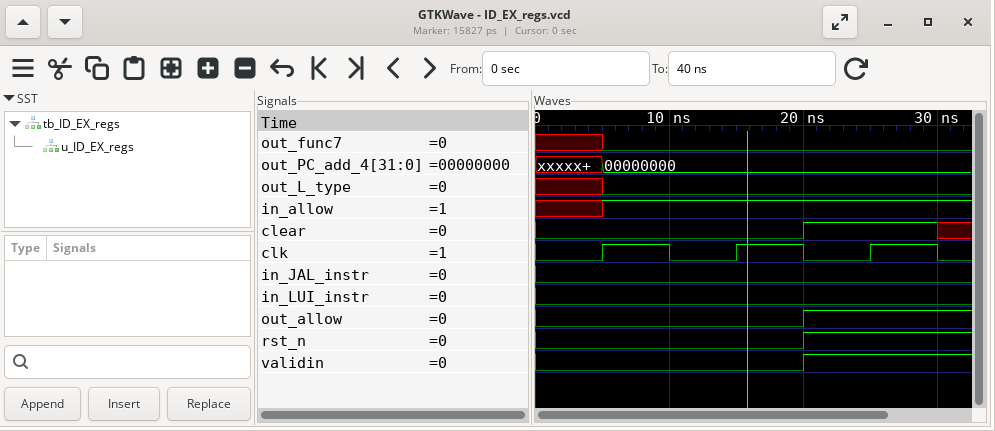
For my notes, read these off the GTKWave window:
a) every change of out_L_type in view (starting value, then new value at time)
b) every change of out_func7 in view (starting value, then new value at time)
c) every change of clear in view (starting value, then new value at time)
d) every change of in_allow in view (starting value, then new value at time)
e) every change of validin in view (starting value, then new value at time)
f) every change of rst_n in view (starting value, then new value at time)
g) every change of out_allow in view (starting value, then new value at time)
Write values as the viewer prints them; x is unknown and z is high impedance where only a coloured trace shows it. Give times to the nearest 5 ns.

x, 0 at 5 ns
x, 0 at 5 ns
0, 1 at 20 ns, x at 30 ns
x, 1 at 5 ns
0, 1 at 20 ns
0, 1 at 20 ns
0, 1 at 20 ns
